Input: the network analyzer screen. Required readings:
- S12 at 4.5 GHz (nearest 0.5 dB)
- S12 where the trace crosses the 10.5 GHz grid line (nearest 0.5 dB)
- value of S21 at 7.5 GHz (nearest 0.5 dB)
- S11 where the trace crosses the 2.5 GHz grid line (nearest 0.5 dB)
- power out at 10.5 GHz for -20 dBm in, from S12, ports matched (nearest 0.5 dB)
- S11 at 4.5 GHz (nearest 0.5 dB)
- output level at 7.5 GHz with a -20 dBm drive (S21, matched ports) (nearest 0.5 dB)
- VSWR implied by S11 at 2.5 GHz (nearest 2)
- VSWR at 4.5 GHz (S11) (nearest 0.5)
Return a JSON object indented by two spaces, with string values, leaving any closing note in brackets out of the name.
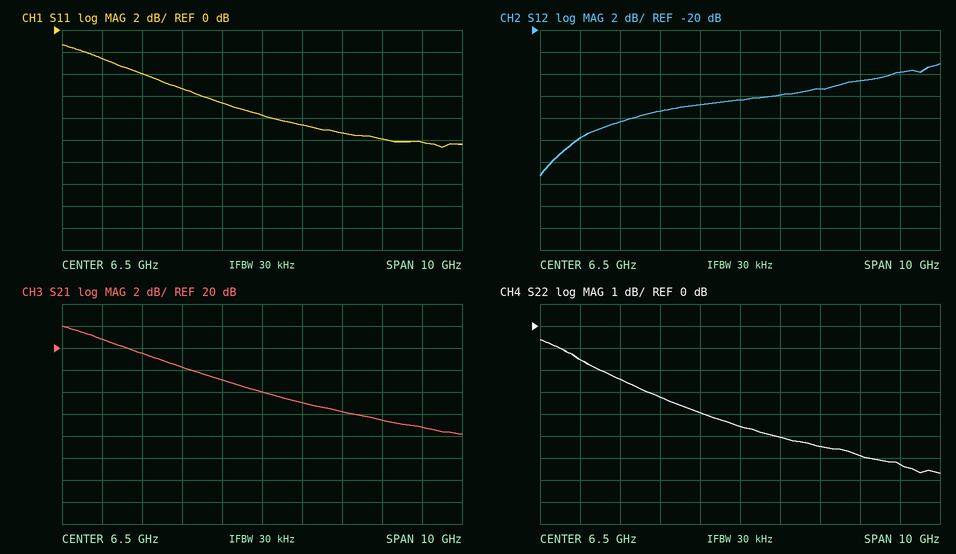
{
  "S12 at 4.5 GHz": "-27.5 dB",
  "S12 where the trace crosses the 10.5 GHz grid line": "-24.0 dB",
  "value of S21 at 7.5 GHz": "15.0 dB",
  "S11 where the trace crosses the 2.5 GHz grid line": "-2.5 dB",
  "power out at 10.5 GHz for -20 dBm in, from S12, ports matched": "-44.0 dBm",
  "S11 at 4.5 GHz": "-5.5 dB",
  "output level at 7.5 GHz with a -20 dBm drive (S21, matched ports)": "-5.0 dBm",
  "VSWR implied by S11 at 2.5 GHz": "6",
  "VSWR at 4.5 GHz (S11)": "3.5"
}
